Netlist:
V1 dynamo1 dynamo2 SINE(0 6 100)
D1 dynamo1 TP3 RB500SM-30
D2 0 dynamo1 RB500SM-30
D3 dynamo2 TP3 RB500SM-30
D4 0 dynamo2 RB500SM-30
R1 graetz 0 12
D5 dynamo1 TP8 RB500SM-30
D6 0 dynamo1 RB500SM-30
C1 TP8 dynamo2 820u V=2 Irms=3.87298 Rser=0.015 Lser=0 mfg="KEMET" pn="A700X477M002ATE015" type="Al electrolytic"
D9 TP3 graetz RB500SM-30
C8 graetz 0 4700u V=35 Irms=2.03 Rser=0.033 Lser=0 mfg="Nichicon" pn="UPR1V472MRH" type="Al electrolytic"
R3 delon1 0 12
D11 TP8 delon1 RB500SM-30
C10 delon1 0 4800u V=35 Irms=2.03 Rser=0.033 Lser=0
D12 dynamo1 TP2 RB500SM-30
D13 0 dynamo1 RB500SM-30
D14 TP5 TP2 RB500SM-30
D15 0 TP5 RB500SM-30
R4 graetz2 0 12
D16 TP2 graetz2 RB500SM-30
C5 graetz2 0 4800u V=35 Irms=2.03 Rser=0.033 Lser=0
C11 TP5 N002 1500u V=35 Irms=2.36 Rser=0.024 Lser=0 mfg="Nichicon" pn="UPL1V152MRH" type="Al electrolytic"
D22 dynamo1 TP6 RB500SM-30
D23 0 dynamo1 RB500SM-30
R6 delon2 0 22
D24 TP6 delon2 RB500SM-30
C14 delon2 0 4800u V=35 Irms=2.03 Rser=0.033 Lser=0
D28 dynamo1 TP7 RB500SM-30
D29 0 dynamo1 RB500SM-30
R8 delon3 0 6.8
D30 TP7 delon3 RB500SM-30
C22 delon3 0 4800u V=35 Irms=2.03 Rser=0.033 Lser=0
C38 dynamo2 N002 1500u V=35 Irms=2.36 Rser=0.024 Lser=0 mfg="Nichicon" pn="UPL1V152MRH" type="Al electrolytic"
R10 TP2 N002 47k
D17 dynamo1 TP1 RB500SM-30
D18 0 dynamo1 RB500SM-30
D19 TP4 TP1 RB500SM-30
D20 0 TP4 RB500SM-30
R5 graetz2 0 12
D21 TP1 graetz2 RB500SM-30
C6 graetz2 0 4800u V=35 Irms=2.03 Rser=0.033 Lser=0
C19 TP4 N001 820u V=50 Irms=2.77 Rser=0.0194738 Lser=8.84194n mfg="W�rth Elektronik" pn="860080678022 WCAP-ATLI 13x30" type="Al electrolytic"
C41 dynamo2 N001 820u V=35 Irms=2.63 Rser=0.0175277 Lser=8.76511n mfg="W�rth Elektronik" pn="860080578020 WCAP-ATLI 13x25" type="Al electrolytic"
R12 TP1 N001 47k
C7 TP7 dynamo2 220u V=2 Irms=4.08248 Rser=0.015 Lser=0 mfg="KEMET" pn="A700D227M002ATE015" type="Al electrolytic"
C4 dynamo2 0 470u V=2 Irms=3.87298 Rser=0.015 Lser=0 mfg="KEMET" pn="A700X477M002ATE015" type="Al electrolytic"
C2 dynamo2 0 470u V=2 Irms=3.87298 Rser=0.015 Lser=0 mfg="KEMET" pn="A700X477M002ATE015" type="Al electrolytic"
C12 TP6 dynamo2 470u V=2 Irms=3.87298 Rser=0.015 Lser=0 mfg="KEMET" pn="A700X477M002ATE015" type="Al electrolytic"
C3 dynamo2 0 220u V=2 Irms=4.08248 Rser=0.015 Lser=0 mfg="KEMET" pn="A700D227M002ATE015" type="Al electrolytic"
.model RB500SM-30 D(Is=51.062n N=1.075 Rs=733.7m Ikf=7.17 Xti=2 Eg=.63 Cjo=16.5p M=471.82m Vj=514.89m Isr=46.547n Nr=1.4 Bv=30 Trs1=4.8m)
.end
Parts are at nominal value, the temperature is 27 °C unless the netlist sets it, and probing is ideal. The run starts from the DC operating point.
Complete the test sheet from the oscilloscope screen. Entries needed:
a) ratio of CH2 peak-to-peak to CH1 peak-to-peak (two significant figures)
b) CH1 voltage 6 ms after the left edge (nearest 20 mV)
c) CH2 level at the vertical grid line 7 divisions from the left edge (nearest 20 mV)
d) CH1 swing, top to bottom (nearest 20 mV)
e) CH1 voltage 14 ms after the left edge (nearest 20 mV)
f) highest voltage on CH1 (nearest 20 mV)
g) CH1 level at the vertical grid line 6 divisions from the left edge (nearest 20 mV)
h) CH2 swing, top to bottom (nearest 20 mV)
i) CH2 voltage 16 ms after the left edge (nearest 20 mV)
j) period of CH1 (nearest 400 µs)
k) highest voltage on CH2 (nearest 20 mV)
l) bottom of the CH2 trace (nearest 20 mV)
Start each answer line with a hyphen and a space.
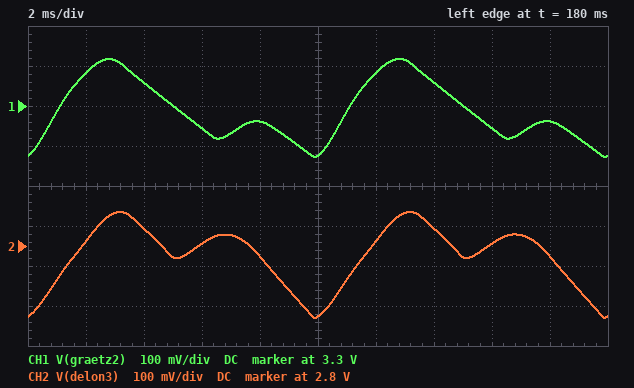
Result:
- 1.1
- 3.24 V
- 2.84 V
- 240 mV
- 3.36 V
- 3.42 V
- 3.38 V
- 260 mV
- 2.80 V
- 10.0 ms
- 2.88 V
- 2.62 V
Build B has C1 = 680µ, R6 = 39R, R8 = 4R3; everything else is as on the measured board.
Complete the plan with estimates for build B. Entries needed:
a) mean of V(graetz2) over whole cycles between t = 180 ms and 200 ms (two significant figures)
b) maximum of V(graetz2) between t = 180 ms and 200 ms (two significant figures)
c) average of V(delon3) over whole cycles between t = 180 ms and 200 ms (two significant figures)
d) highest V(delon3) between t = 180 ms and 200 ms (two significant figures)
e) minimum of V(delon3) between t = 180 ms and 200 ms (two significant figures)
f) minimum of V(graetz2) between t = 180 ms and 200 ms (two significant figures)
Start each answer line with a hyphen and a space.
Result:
- 3.2 V
- 3.3 V
- 2.2 V
- 2.4 V
- 2.0 V
- 3.1 V
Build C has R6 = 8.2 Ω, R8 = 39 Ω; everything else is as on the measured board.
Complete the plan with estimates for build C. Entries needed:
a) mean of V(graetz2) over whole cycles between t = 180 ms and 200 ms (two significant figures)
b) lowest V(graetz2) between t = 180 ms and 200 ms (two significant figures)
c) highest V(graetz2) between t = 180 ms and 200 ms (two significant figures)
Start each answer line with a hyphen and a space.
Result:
- 3.4 V
- 3.3 V
- 3.6 V
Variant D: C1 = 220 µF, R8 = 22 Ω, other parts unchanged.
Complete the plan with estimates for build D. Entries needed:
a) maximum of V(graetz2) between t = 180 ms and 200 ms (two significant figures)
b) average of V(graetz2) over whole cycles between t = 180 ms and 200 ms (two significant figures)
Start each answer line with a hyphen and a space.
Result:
- 3.5 V
- 3.4 V
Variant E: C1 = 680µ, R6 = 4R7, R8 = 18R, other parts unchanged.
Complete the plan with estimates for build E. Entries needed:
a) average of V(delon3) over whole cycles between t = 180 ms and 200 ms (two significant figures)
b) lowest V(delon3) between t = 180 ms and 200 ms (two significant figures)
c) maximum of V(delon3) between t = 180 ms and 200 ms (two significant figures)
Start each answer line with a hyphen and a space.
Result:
- 3.7 V
- 3.6 V
- 3.8 V
